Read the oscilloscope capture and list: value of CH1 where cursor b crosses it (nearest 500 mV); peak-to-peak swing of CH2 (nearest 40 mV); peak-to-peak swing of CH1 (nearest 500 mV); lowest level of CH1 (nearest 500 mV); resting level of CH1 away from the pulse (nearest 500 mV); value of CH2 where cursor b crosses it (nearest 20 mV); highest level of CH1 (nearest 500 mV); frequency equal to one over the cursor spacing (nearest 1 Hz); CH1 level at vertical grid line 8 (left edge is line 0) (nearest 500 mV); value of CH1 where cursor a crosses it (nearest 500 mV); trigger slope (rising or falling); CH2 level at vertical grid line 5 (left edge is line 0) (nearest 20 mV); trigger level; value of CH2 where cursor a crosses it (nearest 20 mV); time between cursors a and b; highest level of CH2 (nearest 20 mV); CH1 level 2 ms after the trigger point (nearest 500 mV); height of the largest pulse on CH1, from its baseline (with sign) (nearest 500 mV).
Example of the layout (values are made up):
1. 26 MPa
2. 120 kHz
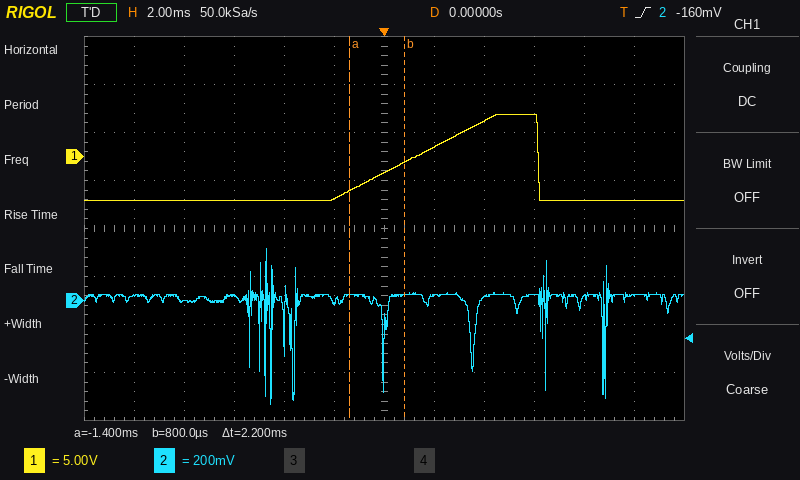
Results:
1. -500 mV
2. 640 mV
3. 9.0 V
4. -4.5 V
5. -4.5 V
6. 20 mV
7. 4.5 V
8. 455 Hz
9. 3.5 V
10. -3.5 V
11. rising
12. 0 mV
13. -160 mV
14. 20 mV
15. 2.2 ms
16. 220 mV
17. 1.0 V
18. +9.0 V
